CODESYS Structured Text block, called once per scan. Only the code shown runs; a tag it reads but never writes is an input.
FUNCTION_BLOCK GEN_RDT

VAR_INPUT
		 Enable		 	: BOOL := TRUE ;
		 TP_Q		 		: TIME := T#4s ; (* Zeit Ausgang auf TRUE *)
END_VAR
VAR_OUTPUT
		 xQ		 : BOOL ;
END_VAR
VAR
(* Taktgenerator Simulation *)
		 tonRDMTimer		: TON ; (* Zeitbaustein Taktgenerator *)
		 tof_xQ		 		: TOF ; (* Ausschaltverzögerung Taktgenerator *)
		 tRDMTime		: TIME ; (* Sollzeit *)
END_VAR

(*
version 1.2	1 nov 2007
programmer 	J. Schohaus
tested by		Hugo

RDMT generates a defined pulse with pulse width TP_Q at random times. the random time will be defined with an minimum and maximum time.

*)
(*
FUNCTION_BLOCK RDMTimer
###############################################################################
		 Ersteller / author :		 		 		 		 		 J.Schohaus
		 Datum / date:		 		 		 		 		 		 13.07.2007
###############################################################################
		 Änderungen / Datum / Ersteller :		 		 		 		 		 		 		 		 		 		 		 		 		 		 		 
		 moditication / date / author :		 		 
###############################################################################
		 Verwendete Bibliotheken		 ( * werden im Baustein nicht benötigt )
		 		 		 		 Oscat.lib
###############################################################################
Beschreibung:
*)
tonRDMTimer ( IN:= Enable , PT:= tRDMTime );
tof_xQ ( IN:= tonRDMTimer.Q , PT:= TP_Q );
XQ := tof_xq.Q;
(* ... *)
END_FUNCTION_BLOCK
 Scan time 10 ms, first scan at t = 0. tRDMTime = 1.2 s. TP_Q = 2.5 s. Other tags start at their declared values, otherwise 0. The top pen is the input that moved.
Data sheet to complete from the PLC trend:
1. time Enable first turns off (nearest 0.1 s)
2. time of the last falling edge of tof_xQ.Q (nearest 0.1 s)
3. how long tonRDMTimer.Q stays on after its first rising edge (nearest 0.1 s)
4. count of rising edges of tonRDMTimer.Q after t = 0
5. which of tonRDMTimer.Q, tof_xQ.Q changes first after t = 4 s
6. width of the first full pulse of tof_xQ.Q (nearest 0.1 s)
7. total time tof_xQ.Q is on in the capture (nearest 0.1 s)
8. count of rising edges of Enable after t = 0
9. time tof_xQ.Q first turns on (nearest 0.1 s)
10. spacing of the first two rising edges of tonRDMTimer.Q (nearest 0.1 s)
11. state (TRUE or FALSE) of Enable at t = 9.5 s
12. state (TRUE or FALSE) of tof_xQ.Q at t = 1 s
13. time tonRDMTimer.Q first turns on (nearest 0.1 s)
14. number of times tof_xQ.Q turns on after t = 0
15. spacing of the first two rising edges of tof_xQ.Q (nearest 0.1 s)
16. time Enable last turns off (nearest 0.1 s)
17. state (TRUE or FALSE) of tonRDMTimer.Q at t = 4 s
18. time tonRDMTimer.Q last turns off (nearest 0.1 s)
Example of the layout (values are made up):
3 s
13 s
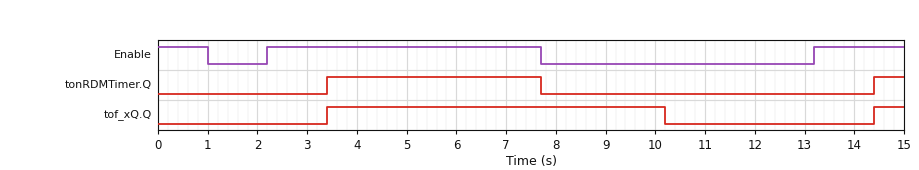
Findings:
1.0 s
10.2 s
4.3 s
2
tonRDMTimer.Q
6.8 s
7.4 s
2
3.4 s
11.0 s
FALSE
FALSE
3.4 s
2
11.0 s
7.7 s
TRUE
7.7 s
